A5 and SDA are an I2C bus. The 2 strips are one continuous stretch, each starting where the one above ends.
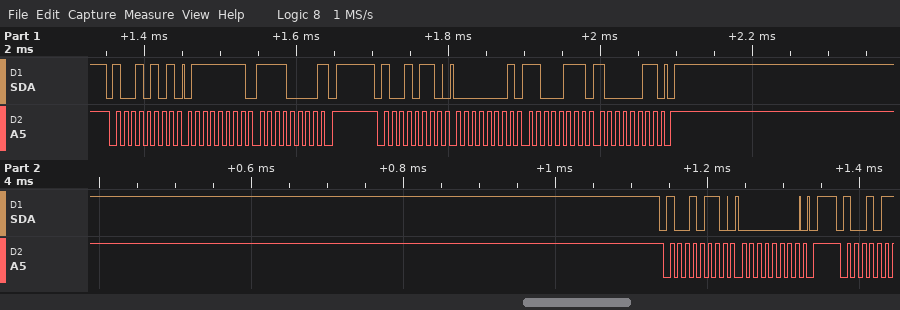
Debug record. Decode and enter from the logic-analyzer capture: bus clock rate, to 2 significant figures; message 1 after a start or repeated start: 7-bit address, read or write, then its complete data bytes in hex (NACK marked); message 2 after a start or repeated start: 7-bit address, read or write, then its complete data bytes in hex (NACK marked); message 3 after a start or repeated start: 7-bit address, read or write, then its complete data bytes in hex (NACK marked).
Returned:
100 kHz
0x4A read: 7F F0 NACK
0x4B write: 01 C7 83
0x4B write: 00
